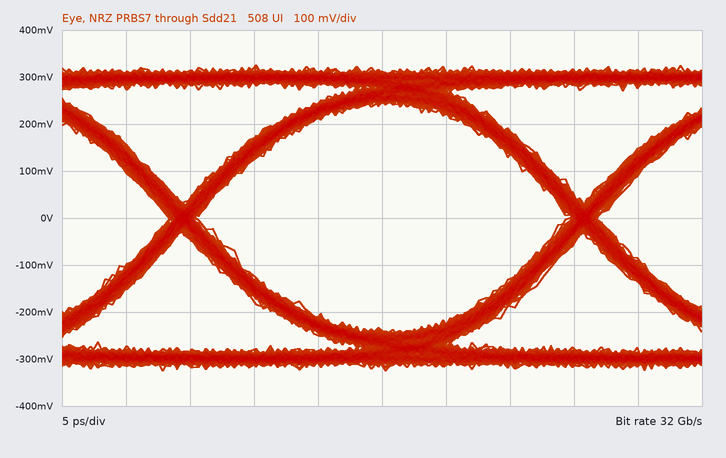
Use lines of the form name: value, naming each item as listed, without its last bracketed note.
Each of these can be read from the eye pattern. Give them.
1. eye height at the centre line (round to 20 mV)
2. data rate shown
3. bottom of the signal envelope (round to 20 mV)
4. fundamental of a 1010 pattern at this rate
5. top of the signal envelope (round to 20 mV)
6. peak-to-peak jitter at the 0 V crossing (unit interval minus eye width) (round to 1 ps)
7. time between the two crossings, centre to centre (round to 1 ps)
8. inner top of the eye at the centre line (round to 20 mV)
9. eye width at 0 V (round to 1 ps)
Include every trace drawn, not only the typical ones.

eye height at the centre line: 480 mV
data rate shown: 32 Gb/s
bottom of the signal envelope: -320 mV
fundamental of a 1010 pattern at this rate: 16 GHz
top of the signal envelope: 320 mV
peak-to-peak jitter at the 0 V crossing (unit interval minus eye width): 2 ps
time between the two crossings, centre to centre: 31 ps
inner top of the eye at the centre line: 240 mV
eye width at 0 V: 29 ps
